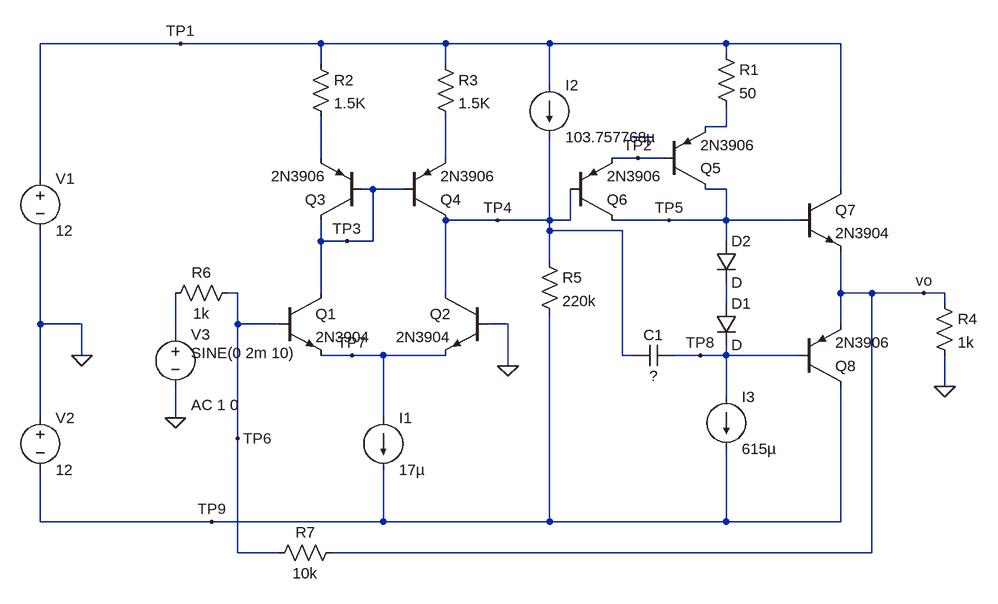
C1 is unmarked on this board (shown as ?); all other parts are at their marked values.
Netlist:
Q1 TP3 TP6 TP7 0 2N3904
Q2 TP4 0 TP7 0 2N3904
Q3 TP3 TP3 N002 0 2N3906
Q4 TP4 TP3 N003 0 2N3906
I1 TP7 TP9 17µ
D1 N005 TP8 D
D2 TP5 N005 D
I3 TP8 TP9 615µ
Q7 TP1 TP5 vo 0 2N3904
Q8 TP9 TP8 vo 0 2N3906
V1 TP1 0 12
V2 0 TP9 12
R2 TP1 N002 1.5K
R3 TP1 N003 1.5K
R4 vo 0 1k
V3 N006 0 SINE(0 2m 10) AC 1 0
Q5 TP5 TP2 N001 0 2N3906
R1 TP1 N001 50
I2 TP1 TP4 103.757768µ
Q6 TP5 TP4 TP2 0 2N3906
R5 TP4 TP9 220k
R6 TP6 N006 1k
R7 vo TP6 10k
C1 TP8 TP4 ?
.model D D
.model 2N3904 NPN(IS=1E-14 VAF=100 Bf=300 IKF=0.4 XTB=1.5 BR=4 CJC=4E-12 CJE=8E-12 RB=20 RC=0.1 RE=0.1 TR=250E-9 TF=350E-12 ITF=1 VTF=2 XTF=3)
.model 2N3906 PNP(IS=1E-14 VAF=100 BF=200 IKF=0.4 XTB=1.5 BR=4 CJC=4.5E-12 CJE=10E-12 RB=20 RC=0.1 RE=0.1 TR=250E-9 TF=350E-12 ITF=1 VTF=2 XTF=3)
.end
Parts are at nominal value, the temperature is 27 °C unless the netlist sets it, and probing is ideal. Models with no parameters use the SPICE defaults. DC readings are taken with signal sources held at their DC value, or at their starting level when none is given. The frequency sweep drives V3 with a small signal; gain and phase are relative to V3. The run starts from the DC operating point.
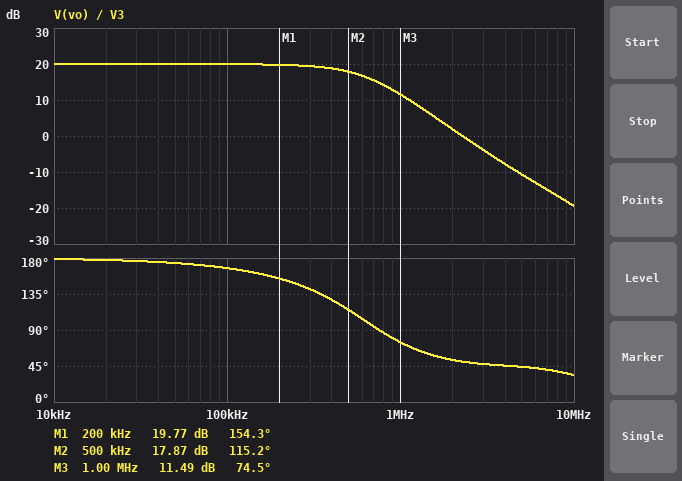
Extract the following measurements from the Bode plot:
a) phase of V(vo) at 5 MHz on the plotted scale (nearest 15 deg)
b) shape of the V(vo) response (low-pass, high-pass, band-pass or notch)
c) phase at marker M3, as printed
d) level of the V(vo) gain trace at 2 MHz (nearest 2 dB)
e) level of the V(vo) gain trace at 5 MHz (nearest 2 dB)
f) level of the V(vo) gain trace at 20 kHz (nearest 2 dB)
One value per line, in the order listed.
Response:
45 deg
low-pass
74.5 deg
2 dB
-10 dB
20 dB
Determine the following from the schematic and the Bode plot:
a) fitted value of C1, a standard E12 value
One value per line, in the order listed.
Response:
8.2 pF
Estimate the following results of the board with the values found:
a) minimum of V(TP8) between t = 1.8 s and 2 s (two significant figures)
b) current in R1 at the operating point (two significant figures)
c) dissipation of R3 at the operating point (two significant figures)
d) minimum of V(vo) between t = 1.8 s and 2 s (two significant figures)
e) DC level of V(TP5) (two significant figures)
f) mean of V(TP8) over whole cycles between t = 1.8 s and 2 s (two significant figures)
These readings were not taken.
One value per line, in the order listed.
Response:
-660 mV
610 µA
110 nW
-20 mV
640 mV
-640 mV
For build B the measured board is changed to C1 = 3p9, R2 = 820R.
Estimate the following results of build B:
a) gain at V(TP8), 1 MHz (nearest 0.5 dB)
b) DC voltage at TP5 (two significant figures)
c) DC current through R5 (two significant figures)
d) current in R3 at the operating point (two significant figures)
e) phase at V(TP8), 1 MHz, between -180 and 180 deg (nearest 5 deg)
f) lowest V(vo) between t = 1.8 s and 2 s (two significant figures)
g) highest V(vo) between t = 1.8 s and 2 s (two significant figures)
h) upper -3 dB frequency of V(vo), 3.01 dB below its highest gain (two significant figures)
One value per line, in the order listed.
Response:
15.0 dB
690 mV
100 µA
7.8 µA
85 deg
26 mV
66 mV
820 kHz
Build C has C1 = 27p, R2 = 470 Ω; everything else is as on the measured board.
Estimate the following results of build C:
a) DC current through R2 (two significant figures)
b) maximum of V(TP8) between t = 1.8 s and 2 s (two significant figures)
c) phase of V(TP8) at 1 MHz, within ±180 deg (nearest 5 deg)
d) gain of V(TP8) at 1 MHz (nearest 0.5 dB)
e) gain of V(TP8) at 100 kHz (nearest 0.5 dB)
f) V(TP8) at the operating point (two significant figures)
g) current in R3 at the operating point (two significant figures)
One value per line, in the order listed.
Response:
9.5 µA
-550 mV
70 deg
1.0 dB
18.5 dB
-570 mV
7.4 µA
